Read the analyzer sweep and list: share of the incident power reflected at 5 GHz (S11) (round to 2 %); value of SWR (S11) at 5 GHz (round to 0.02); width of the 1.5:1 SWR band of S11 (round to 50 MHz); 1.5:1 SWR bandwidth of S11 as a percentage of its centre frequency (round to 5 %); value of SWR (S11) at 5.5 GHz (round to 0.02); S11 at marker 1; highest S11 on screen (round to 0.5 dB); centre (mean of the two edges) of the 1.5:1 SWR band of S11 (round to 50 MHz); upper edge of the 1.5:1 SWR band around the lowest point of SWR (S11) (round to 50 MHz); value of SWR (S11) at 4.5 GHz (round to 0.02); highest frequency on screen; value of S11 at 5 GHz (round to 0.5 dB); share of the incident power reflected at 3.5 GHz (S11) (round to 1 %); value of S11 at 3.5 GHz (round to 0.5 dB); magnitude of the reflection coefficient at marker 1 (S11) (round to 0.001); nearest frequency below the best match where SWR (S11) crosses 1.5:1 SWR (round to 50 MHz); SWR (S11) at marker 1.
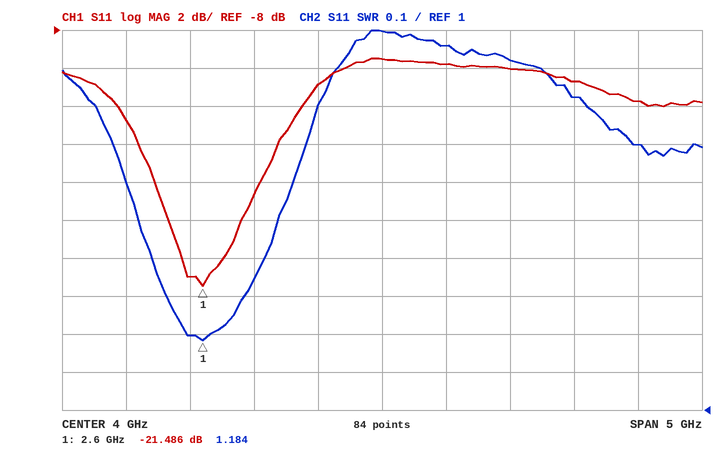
10 %
1.92
1.10 GHz
40 %
1.82
-21.486 dB
-9.5 dB
2.65 GHz
3.20 GHz
1.96
6.5 GHz
-10.0 dB
8 %
-11.0 dB
0.084
2.10 GHz
1.184
